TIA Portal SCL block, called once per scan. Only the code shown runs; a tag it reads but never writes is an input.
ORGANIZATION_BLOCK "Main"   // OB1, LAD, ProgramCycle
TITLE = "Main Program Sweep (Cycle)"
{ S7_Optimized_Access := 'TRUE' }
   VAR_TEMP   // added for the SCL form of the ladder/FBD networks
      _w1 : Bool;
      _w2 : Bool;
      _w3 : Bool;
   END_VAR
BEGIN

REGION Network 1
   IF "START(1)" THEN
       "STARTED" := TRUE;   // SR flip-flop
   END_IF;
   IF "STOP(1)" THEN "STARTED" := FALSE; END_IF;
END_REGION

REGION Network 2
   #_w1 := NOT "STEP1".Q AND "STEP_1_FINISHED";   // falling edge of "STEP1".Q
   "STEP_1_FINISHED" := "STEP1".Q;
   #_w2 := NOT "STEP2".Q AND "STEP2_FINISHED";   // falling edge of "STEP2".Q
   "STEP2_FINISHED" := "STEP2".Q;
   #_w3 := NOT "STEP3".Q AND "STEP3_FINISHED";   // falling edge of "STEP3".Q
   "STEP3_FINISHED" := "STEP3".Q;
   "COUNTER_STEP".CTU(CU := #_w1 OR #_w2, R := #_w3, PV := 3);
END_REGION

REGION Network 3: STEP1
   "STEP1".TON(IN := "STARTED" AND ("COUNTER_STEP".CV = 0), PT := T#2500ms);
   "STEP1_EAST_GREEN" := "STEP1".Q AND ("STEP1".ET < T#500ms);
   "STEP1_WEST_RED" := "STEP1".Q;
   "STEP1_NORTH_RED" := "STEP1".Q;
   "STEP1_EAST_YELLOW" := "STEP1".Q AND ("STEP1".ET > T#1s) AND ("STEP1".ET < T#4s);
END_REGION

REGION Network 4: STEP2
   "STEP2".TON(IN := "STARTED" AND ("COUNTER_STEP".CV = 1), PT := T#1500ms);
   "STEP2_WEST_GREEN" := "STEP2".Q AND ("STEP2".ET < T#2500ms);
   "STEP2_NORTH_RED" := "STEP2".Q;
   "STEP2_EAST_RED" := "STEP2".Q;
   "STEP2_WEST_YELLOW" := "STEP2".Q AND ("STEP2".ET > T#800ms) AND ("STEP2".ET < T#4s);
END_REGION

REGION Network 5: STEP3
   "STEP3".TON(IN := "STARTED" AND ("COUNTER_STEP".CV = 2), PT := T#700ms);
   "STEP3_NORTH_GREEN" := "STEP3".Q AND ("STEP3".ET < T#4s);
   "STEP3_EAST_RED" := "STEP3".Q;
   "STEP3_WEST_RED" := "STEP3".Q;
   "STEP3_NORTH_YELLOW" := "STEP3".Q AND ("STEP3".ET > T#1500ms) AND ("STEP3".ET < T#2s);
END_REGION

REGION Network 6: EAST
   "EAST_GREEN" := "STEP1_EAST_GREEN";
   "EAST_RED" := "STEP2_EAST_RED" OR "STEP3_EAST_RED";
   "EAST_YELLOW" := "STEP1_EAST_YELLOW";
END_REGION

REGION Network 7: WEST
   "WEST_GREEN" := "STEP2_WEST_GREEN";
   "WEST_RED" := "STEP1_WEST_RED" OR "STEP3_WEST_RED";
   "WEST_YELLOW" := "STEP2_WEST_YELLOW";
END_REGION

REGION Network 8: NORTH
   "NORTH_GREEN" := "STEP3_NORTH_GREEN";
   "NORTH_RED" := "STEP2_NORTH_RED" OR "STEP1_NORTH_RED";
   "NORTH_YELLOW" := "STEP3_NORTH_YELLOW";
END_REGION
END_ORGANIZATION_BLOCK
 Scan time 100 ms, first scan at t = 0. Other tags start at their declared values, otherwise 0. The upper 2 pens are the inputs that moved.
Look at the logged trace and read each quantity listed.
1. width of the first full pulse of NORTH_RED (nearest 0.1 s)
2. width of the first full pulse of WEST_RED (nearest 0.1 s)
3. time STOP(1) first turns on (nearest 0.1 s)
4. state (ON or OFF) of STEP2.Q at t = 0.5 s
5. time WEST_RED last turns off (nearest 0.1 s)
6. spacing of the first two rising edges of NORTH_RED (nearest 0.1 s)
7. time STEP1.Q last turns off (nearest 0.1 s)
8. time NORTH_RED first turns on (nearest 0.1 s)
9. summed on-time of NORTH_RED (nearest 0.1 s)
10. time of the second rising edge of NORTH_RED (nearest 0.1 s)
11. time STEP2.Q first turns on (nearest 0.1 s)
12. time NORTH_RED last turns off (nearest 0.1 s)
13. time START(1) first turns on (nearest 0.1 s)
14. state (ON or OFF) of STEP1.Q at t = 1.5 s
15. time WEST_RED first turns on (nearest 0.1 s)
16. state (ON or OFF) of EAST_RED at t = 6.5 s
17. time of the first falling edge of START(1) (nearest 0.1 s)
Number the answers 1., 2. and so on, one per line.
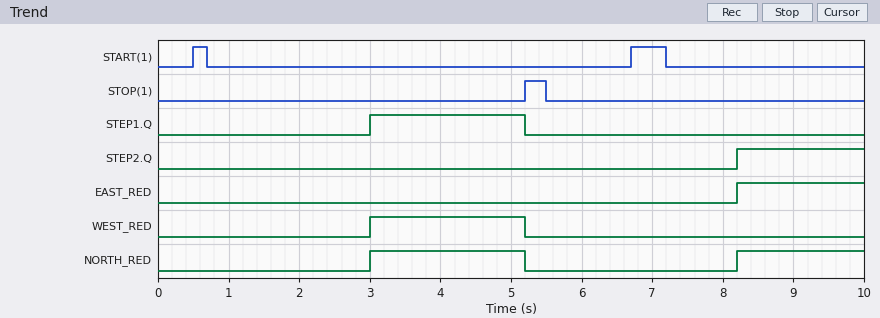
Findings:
1. 2.2 s
2. 2.2 s
3. 5.2 s
4. OFF
5. 5.2 s
6. 5.2 s
7. 5.2 s
8. 3.0 s
9. 4.0 s
10. 8.2 s
11. 8.2 s
12. 5.2 s
13. 0.5 s
14. OFF
15. 3.0 s
16. OFF
17. 0.7 s
